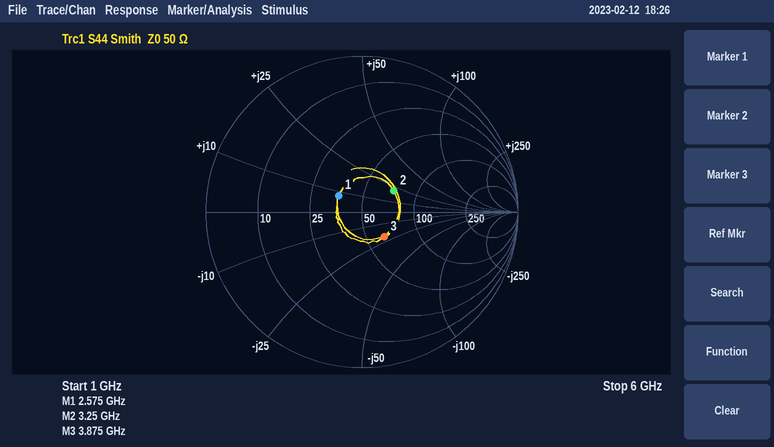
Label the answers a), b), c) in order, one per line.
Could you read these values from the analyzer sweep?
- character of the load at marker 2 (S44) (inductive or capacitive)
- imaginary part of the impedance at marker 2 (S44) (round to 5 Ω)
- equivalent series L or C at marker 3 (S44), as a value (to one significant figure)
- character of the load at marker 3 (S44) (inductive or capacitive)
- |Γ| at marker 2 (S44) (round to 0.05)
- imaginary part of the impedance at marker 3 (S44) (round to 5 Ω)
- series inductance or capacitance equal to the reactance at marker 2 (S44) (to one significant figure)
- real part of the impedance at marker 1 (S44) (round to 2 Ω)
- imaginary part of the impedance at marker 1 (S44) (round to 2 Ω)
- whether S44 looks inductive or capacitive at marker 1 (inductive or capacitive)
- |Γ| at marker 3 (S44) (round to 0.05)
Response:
a) inductive
b) +20 Ω
c) 2 pF
d) capacitive
e) 0.25
f) -20 Ω
g) 1 nH
h) 36 Ω
i) +8 Ω
j) inductive
k) 0.20
